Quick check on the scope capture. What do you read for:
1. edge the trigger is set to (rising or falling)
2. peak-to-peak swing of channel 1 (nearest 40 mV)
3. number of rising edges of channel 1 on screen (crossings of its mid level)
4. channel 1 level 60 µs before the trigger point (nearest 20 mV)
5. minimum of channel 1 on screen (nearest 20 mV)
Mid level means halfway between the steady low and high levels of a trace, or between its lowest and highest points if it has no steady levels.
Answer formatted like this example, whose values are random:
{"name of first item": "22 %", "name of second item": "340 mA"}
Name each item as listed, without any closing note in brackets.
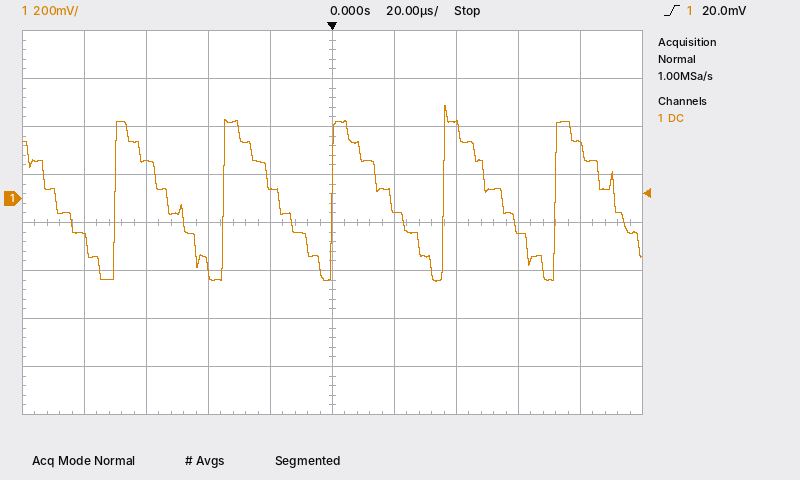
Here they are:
{"edge the trigger is set to": "rising", "peak-to-peak swing of channel 1": "720 mV", "number of rising edges of channel 1 on screen": "5", "channel 1 level 60 µs before the trigger point": "160 mV", "minimum of channel 1 on screen": "-340 mV"}
